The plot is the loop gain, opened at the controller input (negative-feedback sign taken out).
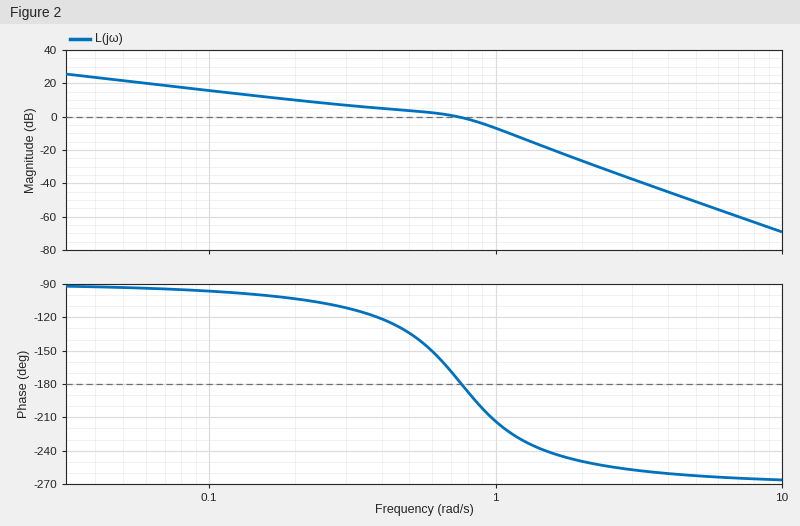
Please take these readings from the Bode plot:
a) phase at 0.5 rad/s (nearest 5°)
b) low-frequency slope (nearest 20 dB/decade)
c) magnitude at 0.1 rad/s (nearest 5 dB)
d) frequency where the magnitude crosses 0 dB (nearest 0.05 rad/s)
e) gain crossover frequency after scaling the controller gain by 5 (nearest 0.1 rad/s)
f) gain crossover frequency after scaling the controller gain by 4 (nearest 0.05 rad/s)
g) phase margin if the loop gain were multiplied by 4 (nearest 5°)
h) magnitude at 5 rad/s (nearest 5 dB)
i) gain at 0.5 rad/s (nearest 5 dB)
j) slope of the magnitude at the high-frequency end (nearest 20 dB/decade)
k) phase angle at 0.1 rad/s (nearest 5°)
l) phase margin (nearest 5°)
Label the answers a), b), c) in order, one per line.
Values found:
a) -135°
b) -20 dB/decade
c) 15 dB
d) 0.75 rad/s
e) 1.3 rad/s
f) 1.20 rad/s
g) -50°
h) -50 dB
i) 5 dB
j) -60 dB/decade
k) -95°
l) 5°
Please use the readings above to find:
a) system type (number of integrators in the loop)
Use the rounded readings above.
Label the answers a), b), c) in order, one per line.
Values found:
a) 1
